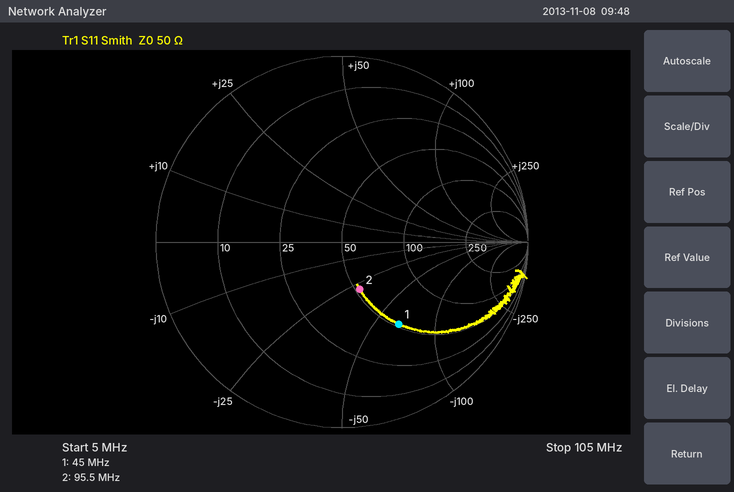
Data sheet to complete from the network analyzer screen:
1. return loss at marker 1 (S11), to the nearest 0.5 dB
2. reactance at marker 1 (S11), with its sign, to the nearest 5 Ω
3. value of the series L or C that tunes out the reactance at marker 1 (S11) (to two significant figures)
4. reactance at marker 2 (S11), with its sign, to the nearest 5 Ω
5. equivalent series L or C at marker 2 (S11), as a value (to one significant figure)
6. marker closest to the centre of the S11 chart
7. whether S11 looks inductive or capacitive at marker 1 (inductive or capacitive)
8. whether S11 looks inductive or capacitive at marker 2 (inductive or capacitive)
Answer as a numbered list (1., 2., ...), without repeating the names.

1. 5.5 dB
2. -65 Ω
3. 230 nH
4. -30 Ω
5. 60 pF
6. marker 2
7. capacitive
8. capacitive
